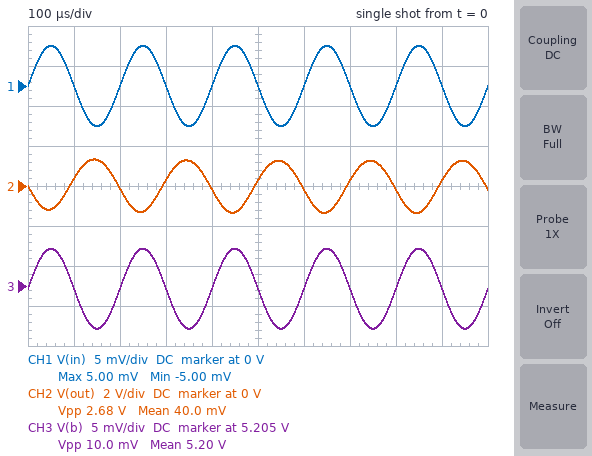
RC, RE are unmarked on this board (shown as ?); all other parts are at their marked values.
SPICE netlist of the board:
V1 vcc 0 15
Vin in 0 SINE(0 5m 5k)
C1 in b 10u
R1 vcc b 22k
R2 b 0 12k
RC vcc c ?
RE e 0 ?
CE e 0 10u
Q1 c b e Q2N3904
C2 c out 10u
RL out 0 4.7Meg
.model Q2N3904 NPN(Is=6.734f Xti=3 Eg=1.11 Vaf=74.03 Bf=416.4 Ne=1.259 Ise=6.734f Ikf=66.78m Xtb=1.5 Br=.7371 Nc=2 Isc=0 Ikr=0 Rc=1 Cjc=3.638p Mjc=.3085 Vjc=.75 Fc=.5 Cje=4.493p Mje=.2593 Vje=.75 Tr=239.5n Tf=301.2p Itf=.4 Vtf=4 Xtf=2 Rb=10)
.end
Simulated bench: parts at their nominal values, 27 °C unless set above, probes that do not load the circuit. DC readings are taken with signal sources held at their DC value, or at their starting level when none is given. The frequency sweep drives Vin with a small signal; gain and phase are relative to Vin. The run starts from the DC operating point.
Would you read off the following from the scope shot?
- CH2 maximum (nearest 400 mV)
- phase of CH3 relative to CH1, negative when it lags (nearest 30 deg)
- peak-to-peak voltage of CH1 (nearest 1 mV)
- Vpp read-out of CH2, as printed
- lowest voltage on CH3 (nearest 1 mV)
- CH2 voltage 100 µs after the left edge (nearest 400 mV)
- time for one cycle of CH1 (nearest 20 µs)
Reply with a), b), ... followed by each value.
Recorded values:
a) 1.2 V
b) 0 deg
c) 10 mV
d) 2.68 V
e) 5.200 V
f) 400 mV
g) 200 µs
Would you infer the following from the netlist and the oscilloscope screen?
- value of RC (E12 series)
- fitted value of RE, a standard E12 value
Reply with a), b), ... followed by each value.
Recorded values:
a) 4.7 kΩ
b) 2.7 kΩ
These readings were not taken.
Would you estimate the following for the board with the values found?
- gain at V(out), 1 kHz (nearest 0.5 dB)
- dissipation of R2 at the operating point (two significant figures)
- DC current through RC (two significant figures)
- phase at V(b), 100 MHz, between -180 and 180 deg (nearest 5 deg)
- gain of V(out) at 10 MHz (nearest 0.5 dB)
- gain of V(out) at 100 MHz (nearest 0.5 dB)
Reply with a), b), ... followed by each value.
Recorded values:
a) 46.0 dB
b) 2.3 mW
c) 1.7 mA
d) 0 deg
e) 45.0 dB
f) 28.0 dB
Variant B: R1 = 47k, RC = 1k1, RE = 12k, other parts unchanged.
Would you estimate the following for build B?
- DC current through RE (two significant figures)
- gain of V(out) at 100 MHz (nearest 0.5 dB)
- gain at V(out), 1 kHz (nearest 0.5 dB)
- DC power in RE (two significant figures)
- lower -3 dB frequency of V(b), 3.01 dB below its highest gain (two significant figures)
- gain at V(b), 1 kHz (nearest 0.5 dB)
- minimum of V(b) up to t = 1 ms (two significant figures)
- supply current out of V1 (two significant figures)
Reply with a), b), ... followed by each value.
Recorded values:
a) 200 µA
b) 15.0 dB
c) 18.5 dB
d) 490 µW
e) 1.7 Hz
f) 0 dB
g) 3.0 V
h) 450 µA
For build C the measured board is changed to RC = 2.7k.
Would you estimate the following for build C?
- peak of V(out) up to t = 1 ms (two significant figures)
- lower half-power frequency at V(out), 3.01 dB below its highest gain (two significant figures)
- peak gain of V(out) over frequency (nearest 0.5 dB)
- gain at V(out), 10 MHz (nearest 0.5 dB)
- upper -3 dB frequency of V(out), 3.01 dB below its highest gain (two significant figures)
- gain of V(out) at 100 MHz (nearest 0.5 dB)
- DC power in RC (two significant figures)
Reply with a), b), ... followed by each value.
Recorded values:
a) 790 mV
b) 960 Hz
c) 44.0 dB
d) 43.0 dB
e) 20 MHz
f) 30.0 dB
g) 7.5 mW
